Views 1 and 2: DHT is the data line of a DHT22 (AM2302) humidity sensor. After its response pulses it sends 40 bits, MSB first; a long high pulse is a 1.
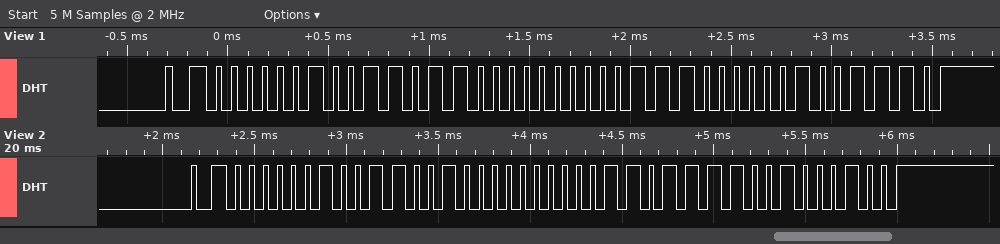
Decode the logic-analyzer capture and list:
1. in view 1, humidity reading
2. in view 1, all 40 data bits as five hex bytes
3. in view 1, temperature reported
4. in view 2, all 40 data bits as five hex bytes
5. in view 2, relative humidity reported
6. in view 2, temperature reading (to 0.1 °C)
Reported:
62.0 %
02 6C 00 E0 4E
22.4 °C
02 64 00 DE 44
61.2 %
22.2 °C
